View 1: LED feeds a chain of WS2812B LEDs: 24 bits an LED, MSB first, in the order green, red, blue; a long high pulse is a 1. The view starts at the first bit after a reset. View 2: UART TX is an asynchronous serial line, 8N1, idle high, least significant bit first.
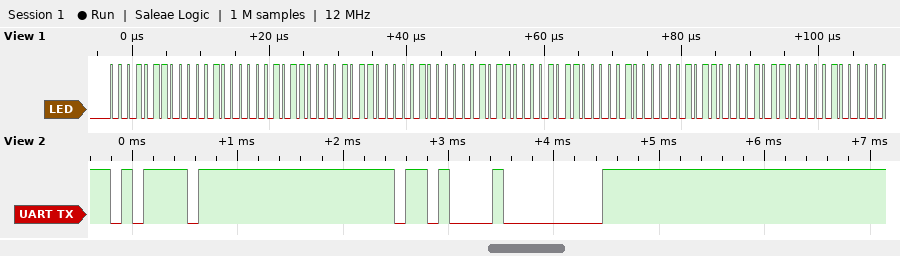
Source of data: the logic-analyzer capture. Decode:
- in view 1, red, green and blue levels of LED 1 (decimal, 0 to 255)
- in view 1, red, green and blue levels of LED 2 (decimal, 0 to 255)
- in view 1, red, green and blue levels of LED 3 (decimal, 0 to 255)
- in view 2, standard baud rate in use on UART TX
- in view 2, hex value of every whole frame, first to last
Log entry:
8, 22, 22
8, 22, 22
8, 22, 22
9600 baud
BD 0B 00
